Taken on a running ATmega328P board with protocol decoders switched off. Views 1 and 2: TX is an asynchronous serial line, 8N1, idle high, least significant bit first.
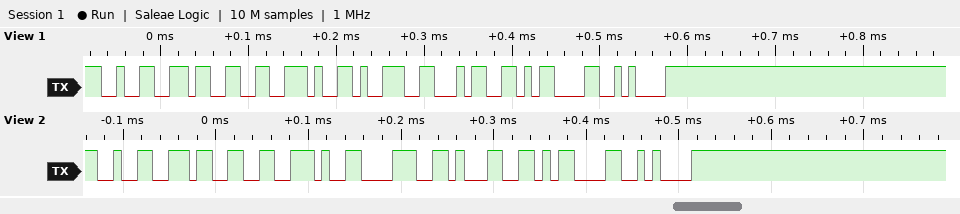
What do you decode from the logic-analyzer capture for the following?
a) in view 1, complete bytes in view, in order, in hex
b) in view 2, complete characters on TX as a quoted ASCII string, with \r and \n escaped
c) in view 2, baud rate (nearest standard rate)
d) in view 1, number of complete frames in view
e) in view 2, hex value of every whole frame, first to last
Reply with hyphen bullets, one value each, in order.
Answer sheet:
- 32 33 2E 39 34 0D 0A
- "23.81\r\n"
- 115200 baud
- 7
- 32 33 2E 38 31 0D 0A
